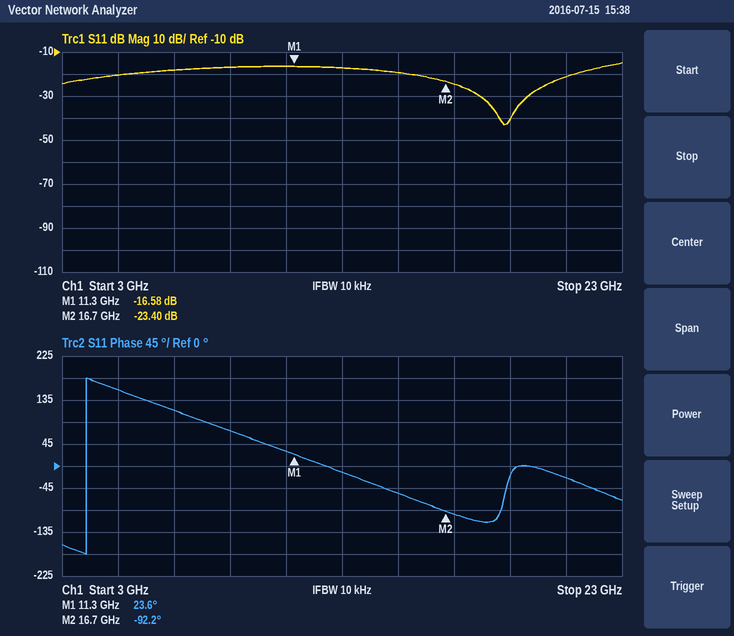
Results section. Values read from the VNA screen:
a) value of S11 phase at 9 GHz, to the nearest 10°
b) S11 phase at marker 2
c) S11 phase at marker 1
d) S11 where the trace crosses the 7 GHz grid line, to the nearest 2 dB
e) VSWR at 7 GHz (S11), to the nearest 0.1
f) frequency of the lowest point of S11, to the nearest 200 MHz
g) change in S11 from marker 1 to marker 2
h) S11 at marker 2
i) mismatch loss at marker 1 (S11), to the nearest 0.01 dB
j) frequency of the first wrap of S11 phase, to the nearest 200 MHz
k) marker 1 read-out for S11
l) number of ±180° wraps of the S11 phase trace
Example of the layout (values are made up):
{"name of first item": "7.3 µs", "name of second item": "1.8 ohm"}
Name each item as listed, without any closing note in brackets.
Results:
{"value of S11 phase at 9 GHz, to the nearest 10°": "70°", "S11 phase at marker 2": "-92.2°", "S11 phase at marker 1": "23.6°", "S11 where the trace crosses the 7 GHz grid line, to the nearest 2 dB": "-18 dB", "VSWR at 7 GHz (S11), to the nearest 0.1": "1.3", "frequency of the lowest point of S11, to the nearest 200 MHz": "18.8 GHz", "change in S11 from marker 1 to marker 2": "-6.82 dB", "S11 at marker 2": "-23.40 dB", "mismatch loss at marker 1 (S11), to the nearest 0.01 dB": "0.10 dB", "frequency of the first wrap of S11 phase, to the nearest 200 MHz": "3.8 GHz", "marker 1 read-out for S11": "-16.58 dB", "number of ±180° wraps of the S11 phase trace": "1"}
